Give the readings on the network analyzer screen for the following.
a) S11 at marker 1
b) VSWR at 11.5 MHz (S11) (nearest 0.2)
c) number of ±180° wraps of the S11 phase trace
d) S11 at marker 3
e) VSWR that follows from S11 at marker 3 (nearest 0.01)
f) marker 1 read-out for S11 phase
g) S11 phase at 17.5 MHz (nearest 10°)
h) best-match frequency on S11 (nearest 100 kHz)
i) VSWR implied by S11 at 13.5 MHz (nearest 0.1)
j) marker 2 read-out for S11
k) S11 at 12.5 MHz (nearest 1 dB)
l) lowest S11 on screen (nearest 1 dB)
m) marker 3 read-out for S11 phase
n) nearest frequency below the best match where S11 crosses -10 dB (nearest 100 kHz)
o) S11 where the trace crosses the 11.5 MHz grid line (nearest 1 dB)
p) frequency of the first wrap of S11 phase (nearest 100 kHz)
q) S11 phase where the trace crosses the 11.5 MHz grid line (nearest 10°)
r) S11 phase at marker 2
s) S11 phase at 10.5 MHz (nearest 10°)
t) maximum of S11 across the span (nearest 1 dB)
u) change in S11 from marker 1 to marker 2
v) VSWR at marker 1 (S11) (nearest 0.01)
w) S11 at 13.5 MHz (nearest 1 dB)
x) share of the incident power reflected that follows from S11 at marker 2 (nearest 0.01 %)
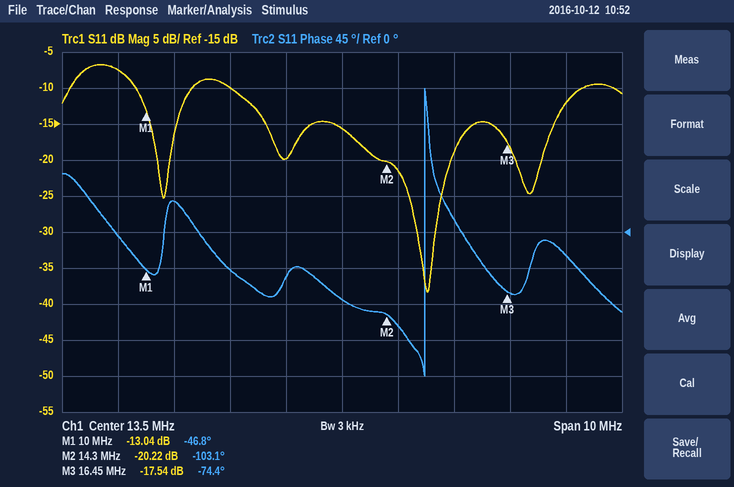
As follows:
-13.04 dB
2.0
1
-17.54 dB
1.31
-46.8°
-30°
15.0 MHz
1.4
-20.22 dB
-20 dB
-38 dB
-74.4°
11.5 MHz
-10 dB
15.0 MHz
-50°
-103.1°
40°
-7 dB
-7.18 dB
1.57
-16 dB
0.95 %
